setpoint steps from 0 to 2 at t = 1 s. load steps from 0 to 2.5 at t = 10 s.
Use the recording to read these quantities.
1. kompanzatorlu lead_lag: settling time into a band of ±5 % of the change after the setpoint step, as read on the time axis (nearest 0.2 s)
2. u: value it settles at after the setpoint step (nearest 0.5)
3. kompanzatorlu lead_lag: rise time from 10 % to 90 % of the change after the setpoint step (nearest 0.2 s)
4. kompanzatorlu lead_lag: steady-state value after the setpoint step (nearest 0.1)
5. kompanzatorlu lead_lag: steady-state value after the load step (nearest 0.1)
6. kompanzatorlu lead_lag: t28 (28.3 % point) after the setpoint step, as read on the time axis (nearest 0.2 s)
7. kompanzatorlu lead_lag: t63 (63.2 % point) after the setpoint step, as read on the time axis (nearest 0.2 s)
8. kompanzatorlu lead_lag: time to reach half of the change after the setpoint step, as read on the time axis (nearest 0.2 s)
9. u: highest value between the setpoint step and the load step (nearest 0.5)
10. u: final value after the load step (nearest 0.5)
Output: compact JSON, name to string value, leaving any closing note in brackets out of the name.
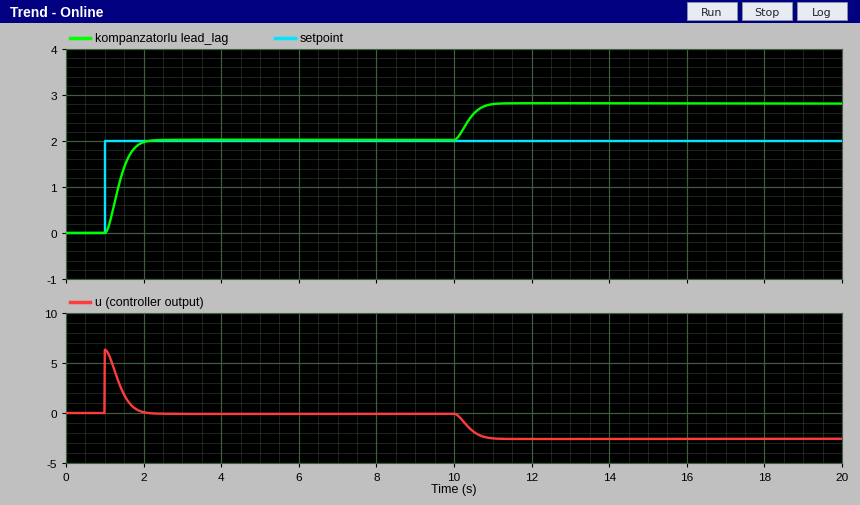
{"kompanzatorlu lead_lag: settling time into a band of ±5 % of the change after the setpoint step, as read on the time axis": "1.8 s", "u: value it settles at after the setpoint step": "0.0", "kompanzatorlu lead_lag: rise time from 10 % to 90 % of the change after the setpoint step": "0.6 s", "kompanzatorlu lead_lag: steady-state value after the setpoint step": "2.0", "kompanzatorlu lead_lag: steady-state value after the load step": "2.8", "kompanzatorlu lead_lag: t28 (28.3 % point) after the setpoint step, as read on the time axis": "1.2 s", "kompanzatorlu lead_lag: t63 (63.2 % point) after the setpoint step, as read on the time axis": "1.4 s", "kompanzatorlu lead_lag: time to reach half of the change after the setpoint step, as read on the time axis": "1.4 s", "u: highest value between the setpoint step and the load step": "6.5", "u: final value after the load step": "-2.5"}
